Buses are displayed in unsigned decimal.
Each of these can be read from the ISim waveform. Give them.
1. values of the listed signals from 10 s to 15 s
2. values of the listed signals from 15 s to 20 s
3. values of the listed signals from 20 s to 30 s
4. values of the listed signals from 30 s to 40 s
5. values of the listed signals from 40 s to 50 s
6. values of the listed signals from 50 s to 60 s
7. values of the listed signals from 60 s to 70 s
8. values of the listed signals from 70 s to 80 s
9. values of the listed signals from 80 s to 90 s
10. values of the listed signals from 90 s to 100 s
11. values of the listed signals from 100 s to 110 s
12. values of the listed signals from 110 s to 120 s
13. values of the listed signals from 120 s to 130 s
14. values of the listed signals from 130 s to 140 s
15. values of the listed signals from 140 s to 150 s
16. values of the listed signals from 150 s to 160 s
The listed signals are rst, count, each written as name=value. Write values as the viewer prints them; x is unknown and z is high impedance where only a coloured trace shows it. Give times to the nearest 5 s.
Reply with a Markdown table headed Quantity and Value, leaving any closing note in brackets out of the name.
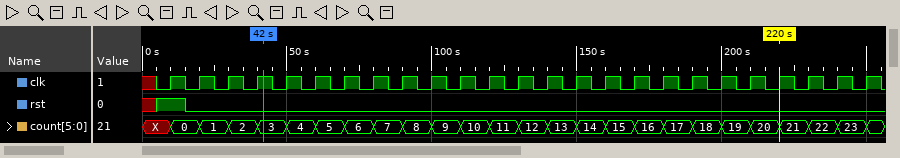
| Quantity | Value |
|---|---|
| values of the listed signals from 10 s to 15 s | rst=1, count=0 |
| values of the listed signals from 15 s to 20 s | rst=0, count=0 |
| values of the listed signals from 20 s to 30 s | rst=0, count=1 |
| values of the listed signals from 30 s to 40 s | rst=0, count=2 |
| values of the listed signals from 40 s to 50 s | rst=0, count=3 |
| values of the listed signals from 50 s to 60 s | rst=0, count=4 |
| values of the listed signals from 60 s to 70 s | rst=0, count=5 |
| values of the listed signals from 70 s to 80 s | rst=0, count=6 |
| values of the listed signals from 80 s to 90 s | rst=0, count=7 |
| values of the listed signals from 90 s to 100 s | rst=0, count=8 |
| values of the listed signals from 100 s to 110 s | rst=0, count=9 |
| values of the listed signals from 110 s to 120 s | rst=0, count=10 |
| values of the listed signals from 120 s to 130 s | rst=0, count=11 |
| values of the listed signals from 130 s to 140 s | rst=0, count=12 |
| values of the listed signals from 140 s to 150 s | rst=0, count=13 |
| values of the listed signals from 150 s to 160 s | rst=0, count=14 |
